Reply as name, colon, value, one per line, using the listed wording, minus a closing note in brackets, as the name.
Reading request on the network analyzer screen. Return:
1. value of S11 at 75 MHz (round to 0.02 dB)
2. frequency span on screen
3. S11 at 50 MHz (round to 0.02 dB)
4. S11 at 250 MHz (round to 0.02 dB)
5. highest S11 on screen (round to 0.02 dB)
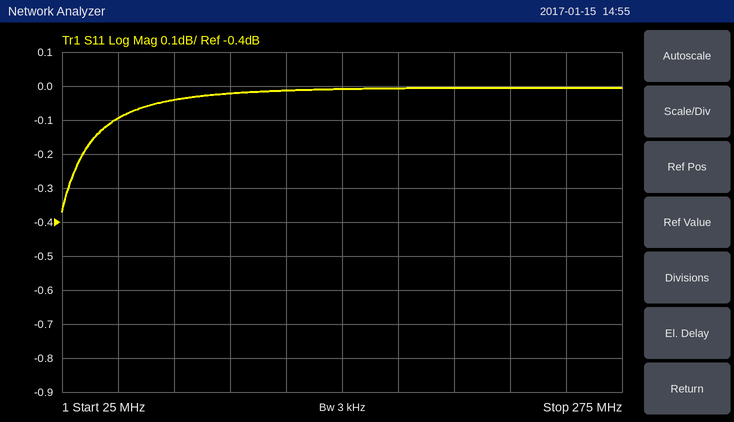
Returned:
value of S11 at 75 MHz: -0.04 dB
frequency span on screen: 250 MHz
S11 at 50 MHz: -0.10 dB
S11 at 250 MHz: 0.00 dB
highest S11 on screen: 0.00 dB
